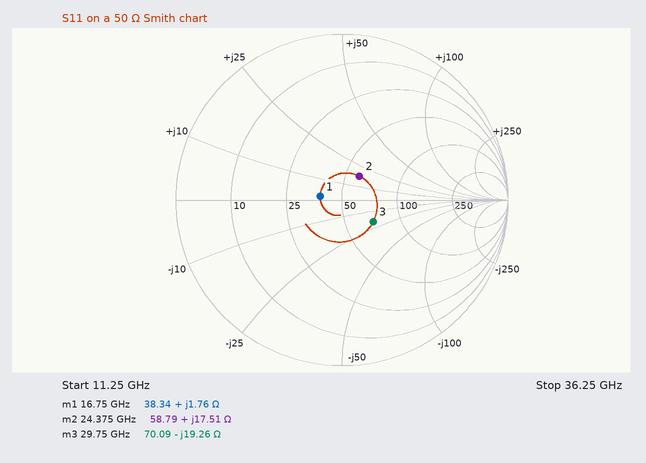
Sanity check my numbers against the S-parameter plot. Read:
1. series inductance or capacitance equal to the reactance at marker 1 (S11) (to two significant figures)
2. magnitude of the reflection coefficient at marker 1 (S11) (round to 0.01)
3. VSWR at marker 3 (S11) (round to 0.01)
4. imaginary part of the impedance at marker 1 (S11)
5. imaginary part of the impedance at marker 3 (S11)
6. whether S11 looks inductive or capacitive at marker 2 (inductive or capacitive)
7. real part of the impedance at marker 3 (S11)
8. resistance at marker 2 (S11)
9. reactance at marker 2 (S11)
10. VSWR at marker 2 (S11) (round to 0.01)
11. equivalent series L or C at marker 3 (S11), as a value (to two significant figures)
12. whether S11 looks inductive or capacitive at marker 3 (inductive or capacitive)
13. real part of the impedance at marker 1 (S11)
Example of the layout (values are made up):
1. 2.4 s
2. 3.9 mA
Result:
1. 17 pH
2. 0.13
3. 1.59
4. +1.76 Ω
5. -19.26 Ω
6. inductive
7. 70.09 Ω
8. 58.79 Ω
9. +17.51 Ω
10. 1.43
11. 280 fF
12. capacitive
13. 38.34 Ω
